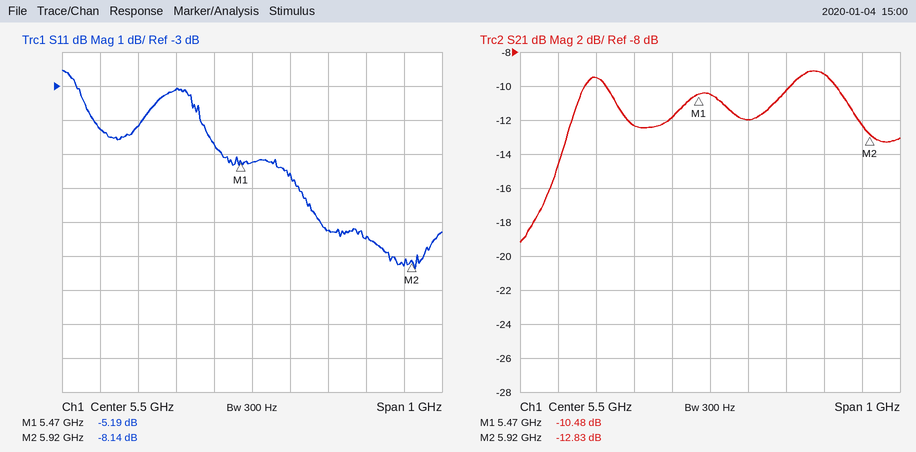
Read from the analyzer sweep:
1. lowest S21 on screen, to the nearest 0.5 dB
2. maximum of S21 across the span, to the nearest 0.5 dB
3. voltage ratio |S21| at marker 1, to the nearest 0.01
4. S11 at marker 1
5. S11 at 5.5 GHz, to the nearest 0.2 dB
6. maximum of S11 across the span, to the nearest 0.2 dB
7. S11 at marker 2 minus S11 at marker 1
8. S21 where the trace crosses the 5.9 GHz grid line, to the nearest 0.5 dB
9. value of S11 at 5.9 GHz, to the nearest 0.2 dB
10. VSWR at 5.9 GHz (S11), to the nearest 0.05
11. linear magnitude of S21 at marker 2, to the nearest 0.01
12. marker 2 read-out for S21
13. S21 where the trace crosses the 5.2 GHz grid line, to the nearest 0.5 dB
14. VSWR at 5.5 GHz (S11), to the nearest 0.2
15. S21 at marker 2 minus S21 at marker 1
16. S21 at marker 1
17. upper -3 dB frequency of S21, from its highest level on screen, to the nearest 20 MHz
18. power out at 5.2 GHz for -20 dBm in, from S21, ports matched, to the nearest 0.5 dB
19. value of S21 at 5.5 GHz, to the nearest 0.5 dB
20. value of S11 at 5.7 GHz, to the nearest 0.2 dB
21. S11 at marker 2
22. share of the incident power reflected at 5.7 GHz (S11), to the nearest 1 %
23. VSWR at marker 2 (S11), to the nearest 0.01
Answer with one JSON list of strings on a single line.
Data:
["-19.0 dB", "-9.0 dB", "0.30", "-5.19 dB", "-5.2 dB", "-2.6 dB", "-2.95 dB", "-12.5 dB", "-8.2 dB", "2.25", "0.23", "-12.83 dB", "-9.5 dB", "3.4", "-2.35 dB", "-10.48 dB", "5.90 GHz", "-29.5 dBm", "-10.5 dB", "-7.2 dB", "-8.14 dB", "19 %", "2.29"]
